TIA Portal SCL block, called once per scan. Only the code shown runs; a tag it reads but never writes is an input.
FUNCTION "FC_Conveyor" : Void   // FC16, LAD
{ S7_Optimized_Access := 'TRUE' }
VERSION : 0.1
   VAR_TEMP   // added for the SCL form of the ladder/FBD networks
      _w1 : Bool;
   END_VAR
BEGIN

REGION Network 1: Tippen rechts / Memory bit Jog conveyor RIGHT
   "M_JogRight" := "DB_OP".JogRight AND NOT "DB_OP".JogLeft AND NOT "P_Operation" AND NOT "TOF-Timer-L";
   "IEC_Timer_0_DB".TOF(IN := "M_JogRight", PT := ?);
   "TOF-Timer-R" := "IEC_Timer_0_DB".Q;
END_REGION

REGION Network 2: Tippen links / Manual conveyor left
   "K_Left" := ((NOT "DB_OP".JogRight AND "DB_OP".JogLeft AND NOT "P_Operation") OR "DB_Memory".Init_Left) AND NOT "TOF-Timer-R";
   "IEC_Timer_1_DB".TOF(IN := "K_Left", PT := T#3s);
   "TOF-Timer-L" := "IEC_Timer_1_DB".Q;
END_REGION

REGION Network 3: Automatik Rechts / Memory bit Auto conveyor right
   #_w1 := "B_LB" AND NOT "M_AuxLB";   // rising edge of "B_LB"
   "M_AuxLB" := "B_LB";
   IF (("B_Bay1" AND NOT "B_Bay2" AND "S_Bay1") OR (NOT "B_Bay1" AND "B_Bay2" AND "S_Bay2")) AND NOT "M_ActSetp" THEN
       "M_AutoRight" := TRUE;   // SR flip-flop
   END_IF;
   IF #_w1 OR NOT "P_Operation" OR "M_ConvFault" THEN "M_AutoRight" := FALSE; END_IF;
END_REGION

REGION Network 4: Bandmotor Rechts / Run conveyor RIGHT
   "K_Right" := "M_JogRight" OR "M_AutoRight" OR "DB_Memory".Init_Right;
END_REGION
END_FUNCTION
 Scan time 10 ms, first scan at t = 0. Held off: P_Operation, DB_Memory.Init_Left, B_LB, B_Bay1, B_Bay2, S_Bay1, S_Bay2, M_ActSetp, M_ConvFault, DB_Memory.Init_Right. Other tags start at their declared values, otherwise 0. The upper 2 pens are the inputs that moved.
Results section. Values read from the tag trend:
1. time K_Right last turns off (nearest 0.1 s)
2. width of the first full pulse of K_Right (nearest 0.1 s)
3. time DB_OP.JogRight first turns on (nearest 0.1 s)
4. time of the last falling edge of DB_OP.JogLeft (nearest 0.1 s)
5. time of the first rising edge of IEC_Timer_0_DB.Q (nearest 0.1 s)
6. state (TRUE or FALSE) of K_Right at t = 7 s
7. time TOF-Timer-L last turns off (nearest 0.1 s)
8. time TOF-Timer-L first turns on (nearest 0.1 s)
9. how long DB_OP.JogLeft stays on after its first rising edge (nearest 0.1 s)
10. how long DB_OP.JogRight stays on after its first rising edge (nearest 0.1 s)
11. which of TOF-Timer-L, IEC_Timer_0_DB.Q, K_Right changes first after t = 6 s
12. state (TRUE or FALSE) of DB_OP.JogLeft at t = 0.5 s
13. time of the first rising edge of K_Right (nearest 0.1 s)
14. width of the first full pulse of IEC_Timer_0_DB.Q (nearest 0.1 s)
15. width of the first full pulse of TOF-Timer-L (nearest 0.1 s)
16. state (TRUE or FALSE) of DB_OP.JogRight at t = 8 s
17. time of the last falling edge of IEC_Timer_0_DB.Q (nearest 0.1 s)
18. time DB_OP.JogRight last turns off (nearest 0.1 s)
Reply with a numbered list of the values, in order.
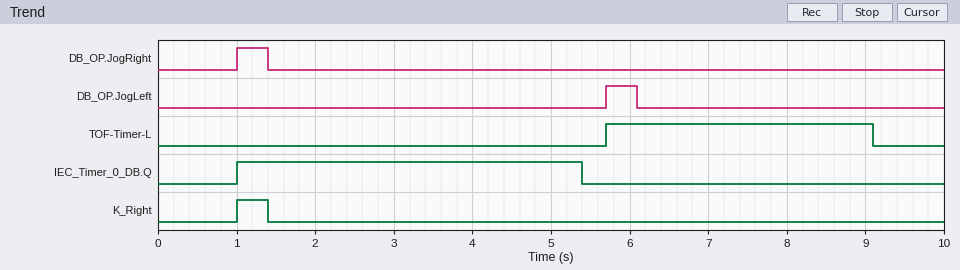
1. 1.4 s
2. 0.4 s
3. 1.0 s
4. 6.1 s
5. 1.0 s
6. FALSE
7. 9.1 s
8. 5.7 s
9. 0.4 s
10. 0.4 s
11. TOF-Timer-L
12. FALSE
13. 1.0 s
14. 4.4 s
15. 3.4 s
16. FALSE
17. 5.4 s
18. 1.4 s
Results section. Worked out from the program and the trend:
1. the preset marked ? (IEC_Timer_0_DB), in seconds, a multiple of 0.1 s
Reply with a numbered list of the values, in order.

1. 4.0 s
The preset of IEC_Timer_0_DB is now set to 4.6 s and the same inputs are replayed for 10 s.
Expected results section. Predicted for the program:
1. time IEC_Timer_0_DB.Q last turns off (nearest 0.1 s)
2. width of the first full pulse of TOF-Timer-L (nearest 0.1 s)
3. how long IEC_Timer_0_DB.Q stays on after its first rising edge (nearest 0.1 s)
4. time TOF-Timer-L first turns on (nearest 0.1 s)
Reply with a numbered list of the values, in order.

1. 6.0 s
2. 3.1 s
3. 5.0 s
4. 6.0 s
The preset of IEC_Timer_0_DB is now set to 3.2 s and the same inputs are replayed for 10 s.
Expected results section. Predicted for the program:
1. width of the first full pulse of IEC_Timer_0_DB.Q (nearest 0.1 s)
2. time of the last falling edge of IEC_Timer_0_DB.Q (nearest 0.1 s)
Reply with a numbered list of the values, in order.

1. 3.6 s
2. 4.6 s
